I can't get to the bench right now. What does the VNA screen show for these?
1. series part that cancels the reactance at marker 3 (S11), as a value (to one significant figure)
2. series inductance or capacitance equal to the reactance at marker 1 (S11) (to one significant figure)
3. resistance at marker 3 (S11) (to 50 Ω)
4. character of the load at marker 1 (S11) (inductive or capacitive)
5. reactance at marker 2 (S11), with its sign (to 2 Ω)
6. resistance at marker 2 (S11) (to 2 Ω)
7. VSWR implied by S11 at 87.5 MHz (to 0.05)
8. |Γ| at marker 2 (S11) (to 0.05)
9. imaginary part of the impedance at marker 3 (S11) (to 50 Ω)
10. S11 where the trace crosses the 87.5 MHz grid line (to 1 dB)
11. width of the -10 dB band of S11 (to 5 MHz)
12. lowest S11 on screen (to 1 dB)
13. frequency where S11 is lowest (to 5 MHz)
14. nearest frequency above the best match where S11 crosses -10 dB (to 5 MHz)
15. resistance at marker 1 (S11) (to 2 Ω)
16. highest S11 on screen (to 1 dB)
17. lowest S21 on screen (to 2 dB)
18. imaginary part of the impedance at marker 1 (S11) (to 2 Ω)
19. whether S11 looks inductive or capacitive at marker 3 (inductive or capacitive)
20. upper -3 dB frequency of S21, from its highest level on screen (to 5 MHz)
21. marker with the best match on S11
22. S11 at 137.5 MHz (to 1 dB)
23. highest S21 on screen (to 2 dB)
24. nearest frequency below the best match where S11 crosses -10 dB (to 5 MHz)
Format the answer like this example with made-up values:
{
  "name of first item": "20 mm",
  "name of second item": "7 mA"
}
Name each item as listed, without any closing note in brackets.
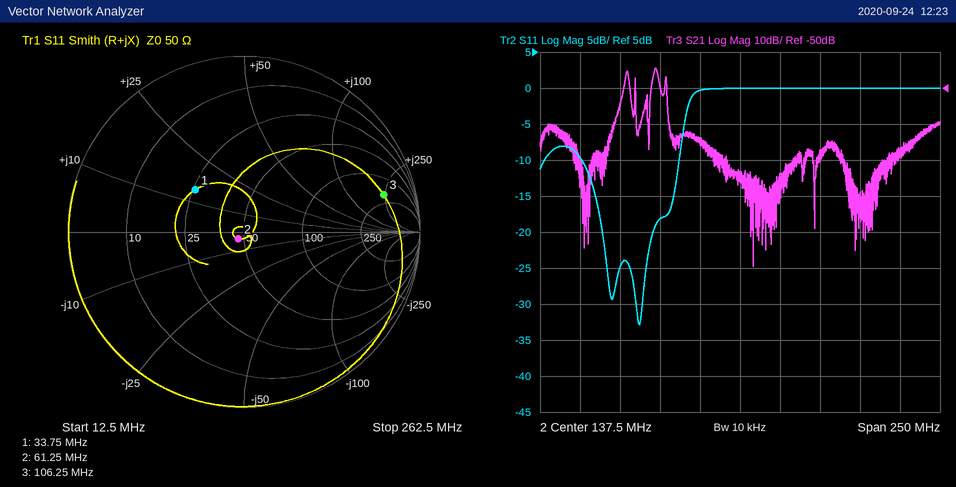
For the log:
{
  "series part that cancels the reactance at marker 3 (S11), as a value": "6 pF",
  "series inductance or capacitance equal to the reactance at marker 1 (S11)": "70 nH",
  "resistance at marker 3 (S11)": "200 Ω",
  "character of the load at marker 1 (S11)": "inductive",
  "reactance at marker 2 (S11), with its sign": "-4 Ω",
  "resistance at marker 2 (S11)": "46 Ω",
  "VSWR implied by S11 at 87.5 MHz": "1.30",
  "|Γ| at marker 2 (S11)": "0.05",
  "imaginary part of the impedance at marker 3 (S11)": "+250 Ω",
  "S11 where the trace crosses the 87.5 MHz grid line": "-18 dB",
  "width of the -10 dB band of S11": "60 MHz",
  "lowest S11 on screen": "-33 dB",
  "frequency where S11 is lowest": "75 MHz",
  "nearest frequency above the best match where S11 crosses -10 dB": "100 MHz",
  "resistance at marker 1 (S11)": "26 Ω",
  "highest S11 on screen": "0 dB",
  "lowest S21 on screen": "-100 dB",
  "imaginary part of the impedance at marker 1 (S11)": "+14 Ω",
  "whether S11 looks inductive or capacitive at marker 3": "inductive",
  "upper -3 dB frequency of S21, from its highest level on screen": "85 MHz",
  "marker with the best match on S11": "marker 2",
  "S11 at 137.5 MHz": "0 dB",
  "highest S21 on screen": "-44 dB",
  "nearest frequency below the best match where S11 crosses -10 dB": "40 MHz"
}
